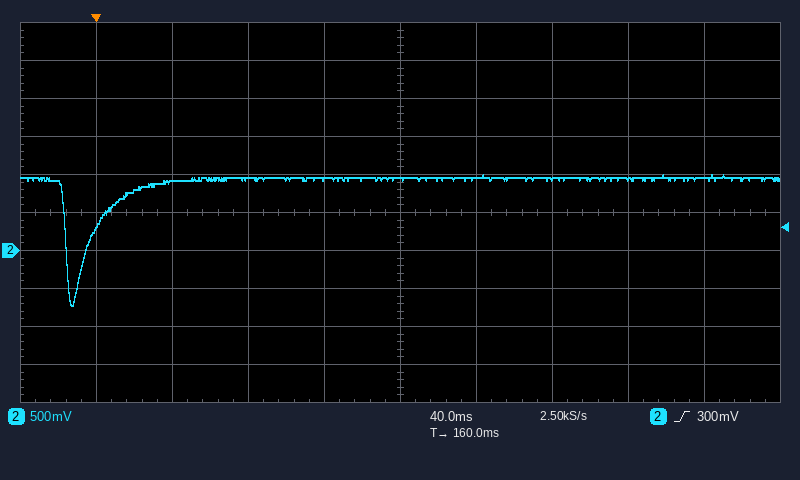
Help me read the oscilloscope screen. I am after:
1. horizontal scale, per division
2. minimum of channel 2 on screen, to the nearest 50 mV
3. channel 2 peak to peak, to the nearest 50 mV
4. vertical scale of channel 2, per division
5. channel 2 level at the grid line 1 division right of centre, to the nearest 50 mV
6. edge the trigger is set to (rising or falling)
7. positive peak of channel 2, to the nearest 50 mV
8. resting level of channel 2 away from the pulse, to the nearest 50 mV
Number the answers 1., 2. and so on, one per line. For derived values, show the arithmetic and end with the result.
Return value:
1. 40 ms
2. -700 mV
3. 1.00 V − (-700 mV) = 1.70 V
4. 500 mV
5. 950 mV
6. rising
7. 1.00 V
8. 950 mV
